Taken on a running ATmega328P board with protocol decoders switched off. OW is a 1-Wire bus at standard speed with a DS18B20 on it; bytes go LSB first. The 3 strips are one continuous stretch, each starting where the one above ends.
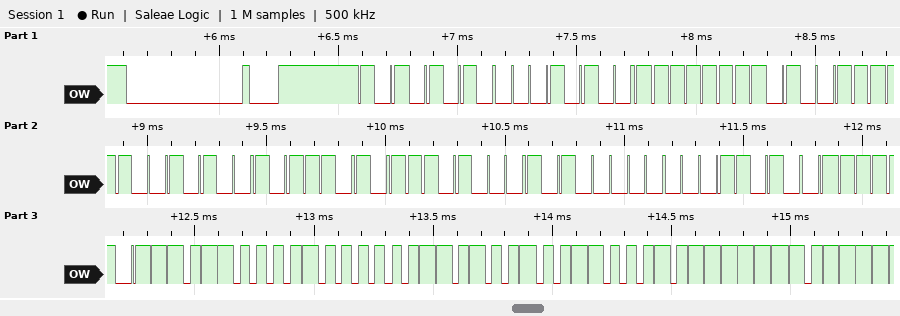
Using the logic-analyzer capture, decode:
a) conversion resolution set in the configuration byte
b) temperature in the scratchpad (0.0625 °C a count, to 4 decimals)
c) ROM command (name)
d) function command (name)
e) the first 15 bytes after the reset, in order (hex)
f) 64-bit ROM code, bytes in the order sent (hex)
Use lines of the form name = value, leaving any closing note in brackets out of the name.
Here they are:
conversion resolution set in the configuration byte = 12 bits
temperature in the scratchpad = 33.6875 °C
ROM command = Match ROM
function command = Read Scratchpad
the first 15 bytes after the reset, in order = 55 28 FF F2 29 5D 17 05 58 BE 1B 02 4B 46 7F
64-bit ROM code, bytes in the order sent = 28 FF F2 29 5D 17 05 58
